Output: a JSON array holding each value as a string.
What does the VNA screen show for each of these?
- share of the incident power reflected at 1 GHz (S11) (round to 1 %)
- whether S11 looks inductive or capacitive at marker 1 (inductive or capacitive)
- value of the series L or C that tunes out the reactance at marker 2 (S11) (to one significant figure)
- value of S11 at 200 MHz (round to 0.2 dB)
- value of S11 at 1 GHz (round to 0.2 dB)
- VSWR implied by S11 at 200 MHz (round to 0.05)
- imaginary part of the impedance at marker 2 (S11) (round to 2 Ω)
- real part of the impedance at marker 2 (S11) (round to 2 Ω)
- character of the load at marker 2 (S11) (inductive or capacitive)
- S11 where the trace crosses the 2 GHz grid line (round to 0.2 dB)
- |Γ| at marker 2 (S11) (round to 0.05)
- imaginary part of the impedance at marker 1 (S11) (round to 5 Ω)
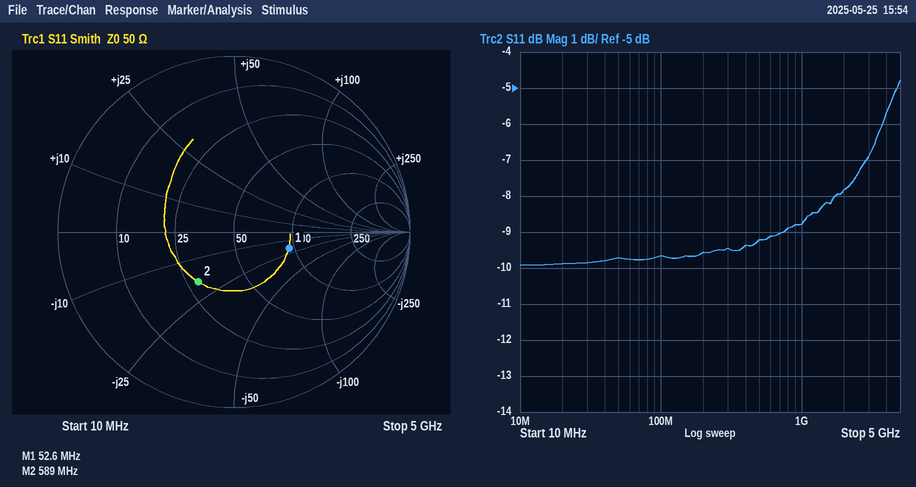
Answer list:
["13 %", "capacitive", "5 nH", "-9.6 dB", "-8.8 dB", "2.00", "-18 Ω", "28 Ω", "capacitive", "-7.8 dB", "0.35", "-20 Ω"]
